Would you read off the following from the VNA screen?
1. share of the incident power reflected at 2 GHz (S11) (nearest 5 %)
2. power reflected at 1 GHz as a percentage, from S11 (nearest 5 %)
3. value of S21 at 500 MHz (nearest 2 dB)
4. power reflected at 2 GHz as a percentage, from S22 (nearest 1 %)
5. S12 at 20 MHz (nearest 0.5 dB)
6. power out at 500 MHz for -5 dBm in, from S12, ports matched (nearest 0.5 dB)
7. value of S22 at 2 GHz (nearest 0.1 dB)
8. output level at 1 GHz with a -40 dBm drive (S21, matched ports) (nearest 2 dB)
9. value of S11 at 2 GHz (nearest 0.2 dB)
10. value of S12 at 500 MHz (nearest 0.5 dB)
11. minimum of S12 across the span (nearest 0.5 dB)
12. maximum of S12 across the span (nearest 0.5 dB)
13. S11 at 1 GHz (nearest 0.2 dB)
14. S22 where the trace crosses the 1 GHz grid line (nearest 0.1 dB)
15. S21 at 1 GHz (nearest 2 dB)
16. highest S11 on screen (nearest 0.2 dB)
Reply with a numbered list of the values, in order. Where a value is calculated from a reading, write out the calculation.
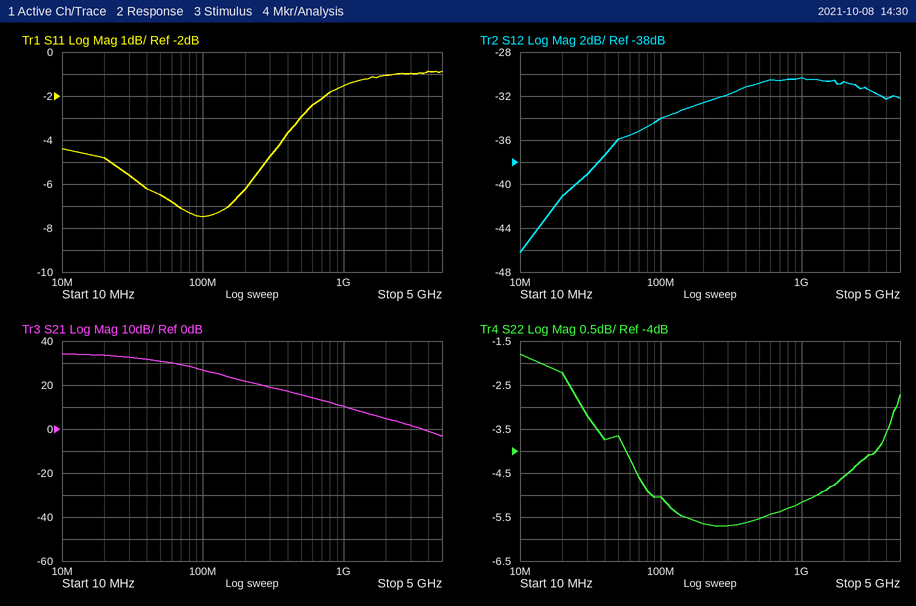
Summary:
1. 10^(-1/10) ≈ 79.4 %, so 80 % to the nearest 5 %
2. 10^(-1.6/10) ≈ 69.2 %, so 70 % to the nearest 5 %
3. 16 dB
4. 10^(-4.6/10) ≈ 35 %
5. -41.0 dB
6. -5 dBm + (-31.0 dB) = -36.0 dBm
7. -4.6 dB
8. -40 dBm + (10 dB) = -30 dBm
9. -1.0 dB
10. -31.0 dB
11. -46.0 dB
12. -30.5 dB
13. -1.6 dB
14. -5.2 dB
15. 10 dB
16. -0.8 dB
